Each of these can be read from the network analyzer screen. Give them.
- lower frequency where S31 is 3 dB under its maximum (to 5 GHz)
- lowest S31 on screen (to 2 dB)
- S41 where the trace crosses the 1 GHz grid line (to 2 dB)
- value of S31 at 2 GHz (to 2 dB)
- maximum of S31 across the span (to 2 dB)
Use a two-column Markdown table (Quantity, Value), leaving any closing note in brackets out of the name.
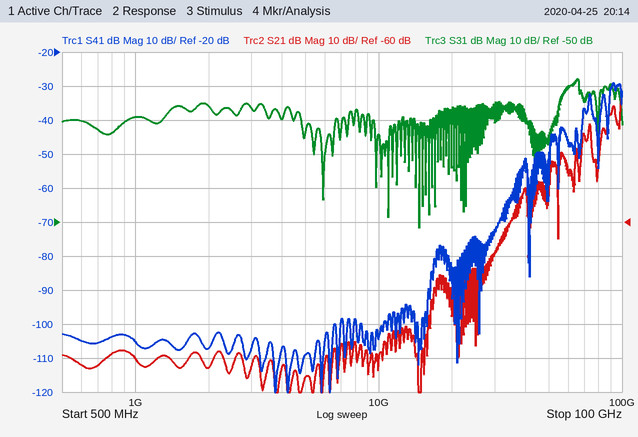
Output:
| Quantity | Value |
|---|---|
| lower frequency where S31 is 3 dB under its maximum | 60 GHz |
| lowest S31 on screen | -52 dB |
| S41 where the trace crosses the 1 GHz grid line | -106 dB |
| value of S31 at 2 GHz | -16 dB |
| maximum of S31 across the span | -8 dB |
